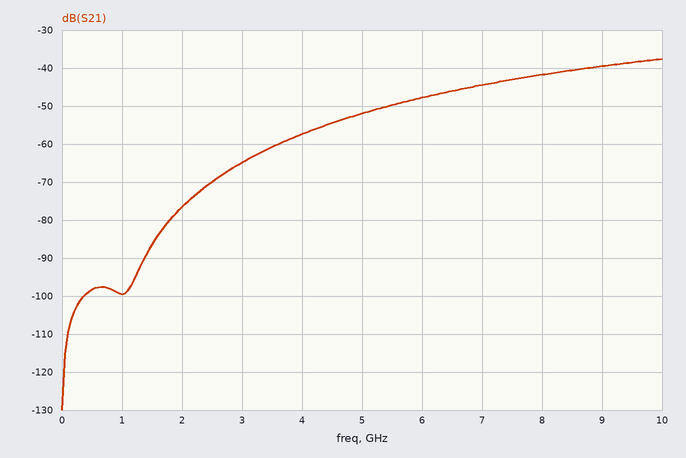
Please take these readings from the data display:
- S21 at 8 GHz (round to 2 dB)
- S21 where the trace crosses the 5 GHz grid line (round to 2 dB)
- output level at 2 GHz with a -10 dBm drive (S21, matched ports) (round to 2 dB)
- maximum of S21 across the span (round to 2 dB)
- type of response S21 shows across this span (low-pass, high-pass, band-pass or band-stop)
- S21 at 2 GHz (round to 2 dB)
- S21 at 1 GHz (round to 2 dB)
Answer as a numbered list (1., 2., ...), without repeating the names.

1. -42 dB
2. -52 dB
3. -86 dBm
4. -38 dB
5. high-pass
6. -76 dB
7. -100 dB
